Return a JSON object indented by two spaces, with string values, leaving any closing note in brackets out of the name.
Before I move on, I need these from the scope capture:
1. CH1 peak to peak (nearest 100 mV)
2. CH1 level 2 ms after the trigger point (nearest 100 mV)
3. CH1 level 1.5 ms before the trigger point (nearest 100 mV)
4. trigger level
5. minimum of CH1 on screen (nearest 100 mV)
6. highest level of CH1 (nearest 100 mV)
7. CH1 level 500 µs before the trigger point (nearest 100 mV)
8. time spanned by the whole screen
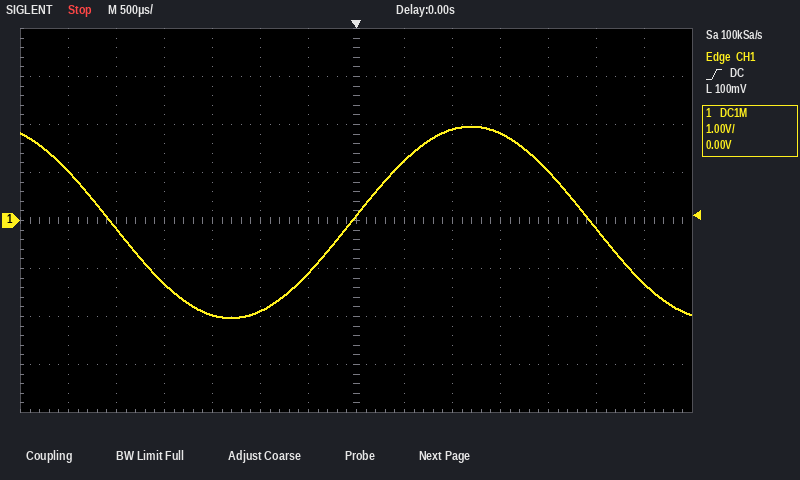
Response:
{
  "CH1 peak to peak": "4.0 V",
  "CH1 level 2 ms after the trigger point": "1.0 V",
  "CH1 level 1.5 ms before the trigger point": "-2.0 V",
  "trigger level": "100 mV",
  "minimum of CH1 on screen": "-2.0 V",
  "highest level of CH1": "2.0 V",
  "CH1 level 500 µs before the trigger point": "-1.1 V",
  "time spanned by the whole screen": "7 ms"
}
